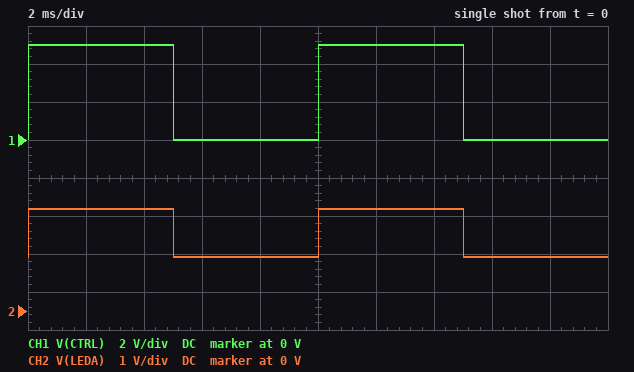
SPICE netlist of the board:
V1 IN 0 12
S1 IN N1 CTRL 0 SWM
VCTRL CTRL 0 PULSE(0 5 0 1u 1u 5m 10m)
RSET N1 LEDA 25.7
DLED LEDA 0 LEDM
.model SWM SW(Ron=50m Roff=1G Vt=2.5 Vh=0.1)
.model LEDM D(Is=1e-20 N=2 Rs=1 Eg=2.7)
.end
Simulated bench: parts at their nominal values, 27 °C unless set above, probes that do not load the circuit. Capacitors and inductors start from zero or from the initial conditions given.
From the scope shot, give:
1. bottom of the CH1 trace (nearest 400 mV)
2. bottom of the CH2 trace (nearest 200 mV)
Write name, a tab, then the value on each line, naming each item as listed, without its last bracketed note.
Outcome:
bottom of the CH1 trace	0 V
bottom of the CH2 trace	1.4 V
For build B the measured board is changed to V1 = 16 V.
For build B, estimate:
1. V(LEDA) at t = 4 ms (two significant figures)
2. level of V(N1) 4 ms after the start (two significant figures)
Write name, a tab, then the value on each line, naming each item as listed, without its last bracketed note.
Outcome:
V(LEDA) at t = 4 ms	2.9 V
level of V(N1) 4 ms after the start	16 V
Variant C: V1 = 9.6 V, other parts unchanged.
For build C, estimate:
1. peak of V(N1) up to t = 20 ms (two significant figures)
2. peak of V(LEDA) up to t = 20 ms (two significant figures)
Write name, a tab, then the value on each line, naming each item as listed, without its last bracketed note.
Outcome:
peak of V(N1) up to t = 20 ms	9.6 V
peak of V(LEDA) up to t = 20 ms	2.6 V
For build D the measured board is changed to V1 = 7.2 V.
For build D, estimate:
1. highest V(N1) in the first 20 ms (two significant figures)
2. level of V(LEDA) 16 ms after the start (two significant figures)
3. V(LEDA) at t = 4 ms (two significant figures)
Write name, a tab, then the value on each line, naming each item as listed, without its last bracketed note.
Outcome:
highest V(N1) in the first 20 ms	7.2 V
level of V(LEDA) 16 ms after the start	1.4 V
V(LEDA) at t = 4 ms	2.5 V
